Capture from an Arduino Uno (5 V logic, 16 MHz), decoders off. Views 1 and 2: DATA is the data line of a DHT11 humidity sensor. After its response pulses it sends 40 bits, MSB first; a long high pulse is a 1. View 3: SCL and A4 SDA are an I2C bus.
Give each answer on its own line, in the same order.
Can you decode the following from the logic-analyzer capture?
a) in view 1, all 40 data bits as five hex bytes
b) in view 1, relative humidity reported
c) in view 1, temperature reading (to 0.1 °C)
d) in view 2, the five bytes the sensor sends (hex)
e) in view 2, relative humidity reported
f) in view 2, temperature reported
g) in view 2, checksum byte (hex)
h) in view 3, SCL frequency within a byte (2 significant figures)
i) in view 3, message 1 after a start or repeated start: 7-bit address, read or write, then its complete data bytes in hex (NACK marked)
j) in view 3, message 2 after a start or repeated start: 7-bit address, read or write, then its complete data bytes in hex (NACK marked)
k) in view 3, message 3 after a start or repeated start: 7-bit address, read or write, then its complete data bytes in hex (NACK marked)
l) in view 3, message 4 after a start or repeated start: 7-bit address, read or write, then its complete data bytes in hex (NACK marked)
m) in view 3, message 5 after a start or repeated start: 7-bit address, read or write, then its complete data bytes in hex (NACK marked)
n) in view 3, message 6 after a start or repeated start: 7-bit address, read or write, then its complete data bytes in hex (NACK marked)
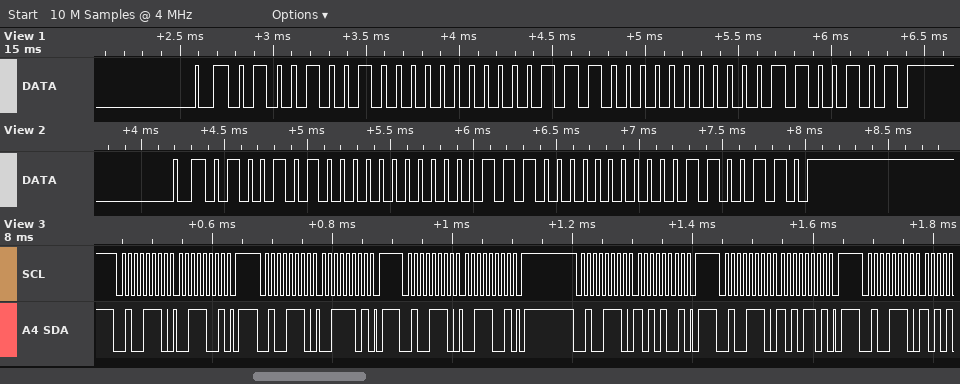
49 00 1C 00 65
73 %
28.0 °C
4A 00 1C 00 66
74 %
28.0 °C
0x66
100 kHz
0x27 write: 39
0x27 write: 3D
0x27 write: 39
0x27 write: A9
0x27 write: AD
0x27 write
